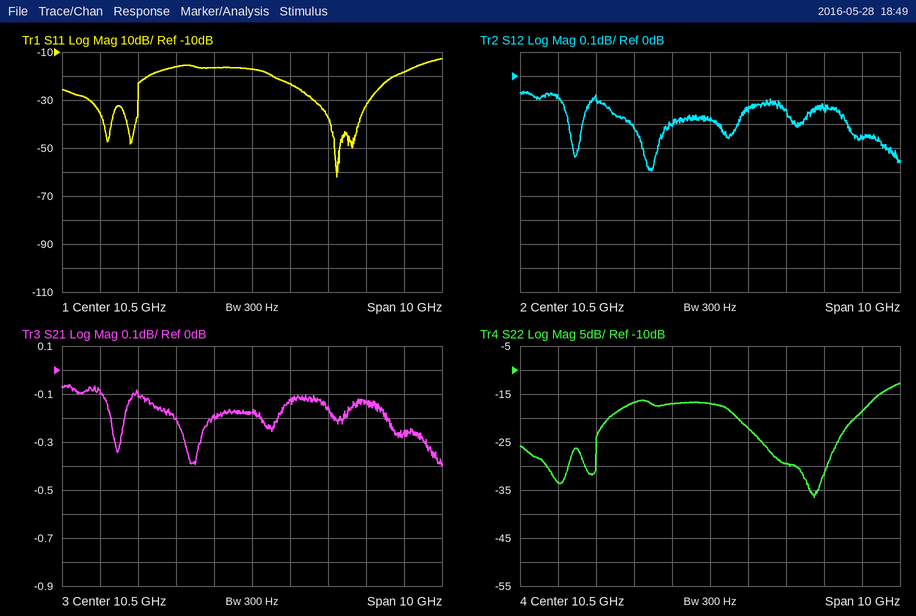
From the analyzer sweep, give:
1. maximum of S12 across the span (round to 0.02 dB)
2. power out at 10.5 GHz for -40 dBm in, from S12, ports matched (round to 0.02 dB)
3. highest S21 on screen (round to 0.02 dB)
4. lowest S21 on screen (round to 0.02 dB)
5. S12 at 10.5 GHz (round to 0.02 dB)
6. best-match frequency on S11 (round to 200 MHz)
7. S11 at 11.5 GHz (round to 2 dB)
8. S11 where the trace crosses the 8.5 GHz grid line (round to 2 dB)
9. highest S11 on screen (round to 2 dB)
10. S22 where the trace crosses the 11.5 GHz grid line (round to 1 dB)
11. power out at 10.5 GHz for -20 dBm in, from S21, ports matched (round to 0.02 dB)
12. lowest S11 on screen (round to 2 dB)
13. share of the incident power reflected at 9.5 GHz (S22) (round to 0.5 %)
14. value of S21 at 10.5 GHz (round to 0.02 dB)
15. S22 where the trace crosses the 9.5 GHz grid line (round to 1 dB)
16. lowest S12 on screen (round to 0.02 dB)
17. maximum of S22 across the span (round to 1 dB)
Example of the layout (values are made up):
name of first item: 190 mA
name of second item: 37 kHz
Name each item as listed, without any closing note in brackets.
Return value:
maximum of S12 across the span: -0.06 dB
power out at 10.5 GHz for -40 dBm in, from S12, ports matched: -40.18 dBm
highest S21 on screen: -0.06 dB
lowest S21 on screen: -0.40 dB
S12 at 10.5 GHz: -0.18 dB
best-match frequency on S11: 12.8 GHz
S11 at 11.5 GHz: -24 dB
S11 where the trace crosses the 8.5 GHz grid line: -16 dB
highest S11 on screen: -12 dB
S22 where the trace crosses the 11.5 GHz grid line: -22 dB
power out at 10.5 GHz for -20 dBm in, from S21, ports matched: -20.18 dBm
lowest S11 on screen: -62 dB
share of the incident power reflected at 9.5 GHz (S22): 2.0 %
value of S21 at 10.5 GHz: -0.18 dB
S22 where the trace crosses the 9.5 GHz grid line: -17 dB
lowest S12 on screen: -0.40 dB
maximum of S22 across the span: -13 dB
